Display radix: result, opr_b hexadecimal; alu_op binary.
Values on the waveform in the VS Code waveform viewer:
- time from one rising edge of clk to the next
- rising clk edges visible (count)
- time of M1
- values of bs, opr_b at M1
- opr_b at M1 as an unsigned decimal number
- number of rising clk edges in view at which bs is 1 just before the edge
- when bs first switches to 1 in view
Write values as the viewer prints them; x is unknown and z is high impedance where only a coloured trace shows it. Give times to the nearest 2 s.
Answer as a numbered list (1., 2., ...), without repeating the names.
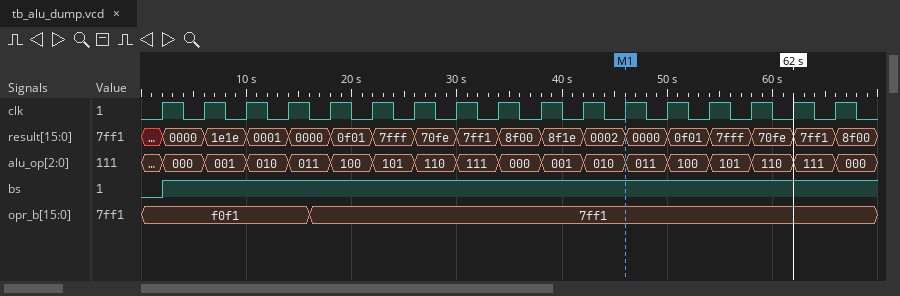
1. 4 s
2. 17
3. 46 s
4. bs=1, opr_b=7ff1
5. 32753
6. 16
7. 2 s
